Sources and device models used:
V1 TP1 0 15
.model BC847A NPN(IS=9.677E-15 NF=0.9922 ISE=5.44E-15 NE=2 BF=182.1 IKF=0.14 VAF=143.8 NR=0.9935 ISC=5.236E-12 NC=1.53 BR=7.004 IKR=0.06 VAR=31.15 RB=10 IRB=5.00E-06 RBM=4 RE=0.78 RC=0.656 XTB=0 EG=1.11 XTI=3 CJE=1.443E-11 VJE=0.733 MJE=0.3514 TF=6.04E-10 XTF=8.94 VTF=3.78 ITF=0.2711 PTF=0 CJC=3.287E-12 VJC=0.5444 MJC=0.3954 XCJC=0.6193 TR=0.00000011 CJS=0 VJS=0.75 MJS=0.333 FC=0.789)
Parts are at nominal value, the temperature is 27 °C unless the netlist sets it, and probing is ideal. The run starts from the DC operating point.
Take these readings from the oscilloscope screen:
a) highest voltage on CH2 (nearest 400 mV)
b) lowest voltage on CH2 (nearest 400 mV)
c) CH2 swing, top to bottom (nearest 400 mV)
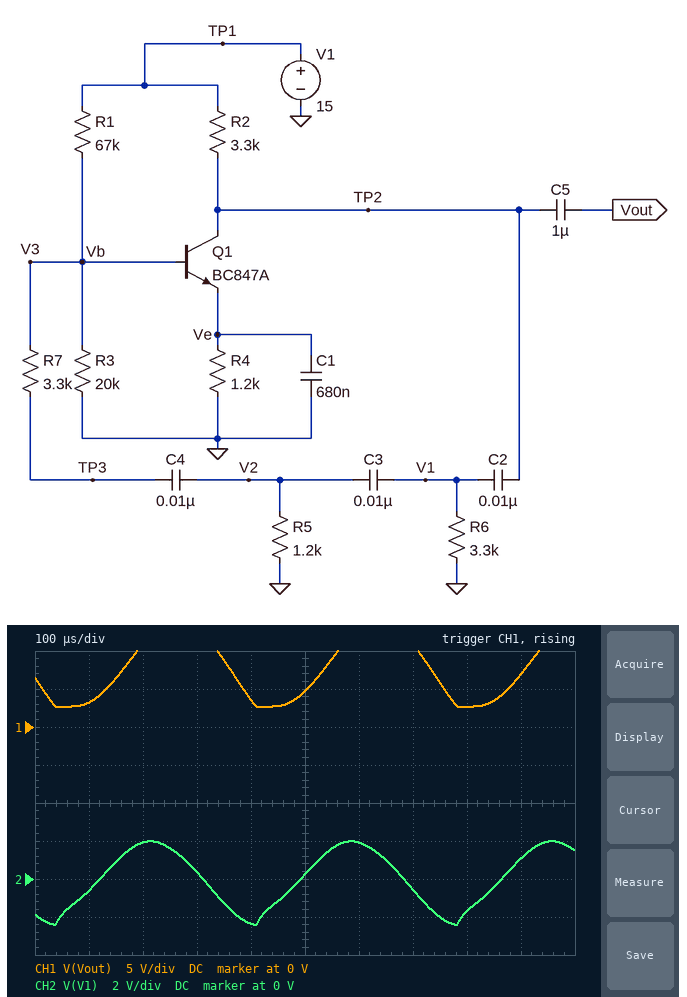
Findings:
2.0 V
-2.4 V
4.4 V
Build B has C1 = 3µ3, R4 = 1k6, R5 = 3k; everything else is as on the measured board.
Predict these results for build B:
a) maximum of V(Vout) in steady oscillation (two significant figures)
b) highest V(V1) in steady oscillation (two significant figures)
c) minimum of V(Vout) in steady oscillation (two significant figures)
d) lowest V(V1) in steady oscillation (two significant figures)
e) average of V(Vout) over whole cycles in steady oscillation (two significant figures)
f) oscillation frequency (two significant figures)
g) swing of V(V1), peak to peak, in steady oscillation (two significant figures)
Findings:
15 V
1.9 V
3.1 V
-1.3 V
9.5 V
1.3 kHz
3.3 V
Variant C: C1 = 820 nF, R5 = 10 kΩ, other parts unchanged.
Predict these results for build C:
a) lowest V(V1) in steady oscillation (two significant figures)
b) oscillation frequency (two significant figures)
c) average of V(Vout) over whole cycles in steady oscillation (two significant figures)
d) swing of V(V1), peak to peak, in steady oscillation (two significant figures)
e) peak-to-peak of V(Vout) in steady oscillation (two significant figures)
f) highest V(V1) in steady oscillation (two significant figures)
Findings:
-2.1 V
1.4 kHz
8.3 V
3.5 V
12 V
1.4 V
